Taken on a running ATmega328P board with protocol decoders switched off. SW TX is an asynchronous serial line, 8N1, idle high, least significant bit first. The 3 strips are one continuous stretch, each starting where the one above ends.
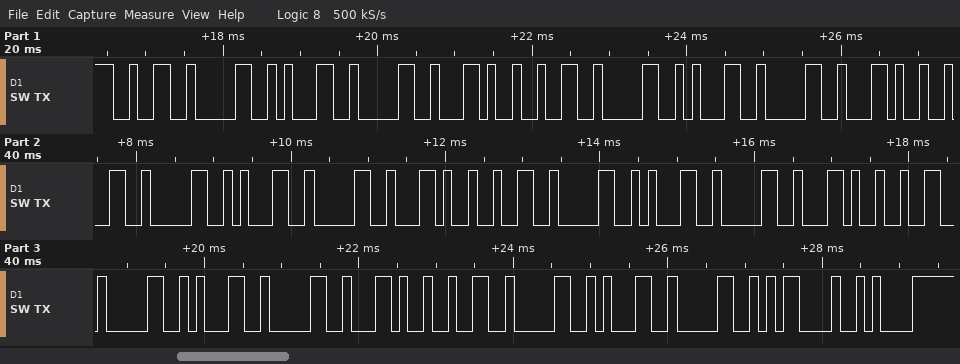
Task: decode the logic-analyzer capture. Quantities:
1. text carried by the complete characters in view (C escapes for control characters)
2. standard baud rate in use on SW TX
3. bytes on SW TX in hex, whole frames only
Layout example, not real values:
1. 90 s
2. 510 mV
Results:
1. "2010,2010,2010,2010,2010,2010\r\n"
2. 9600 baud
3. 0x32 0x30 0x31 0x30 0x2C 0x32 0x30 0x31 0x30 0x2C 0x32 0x30 0x31 0x30 0x2C 0x32 0x30 0x31 0x30 0x2C 0x32 0x30 0x31 0x30 0x2C 0x32 0x30 0x31 0x30 0x0D 0x0A
